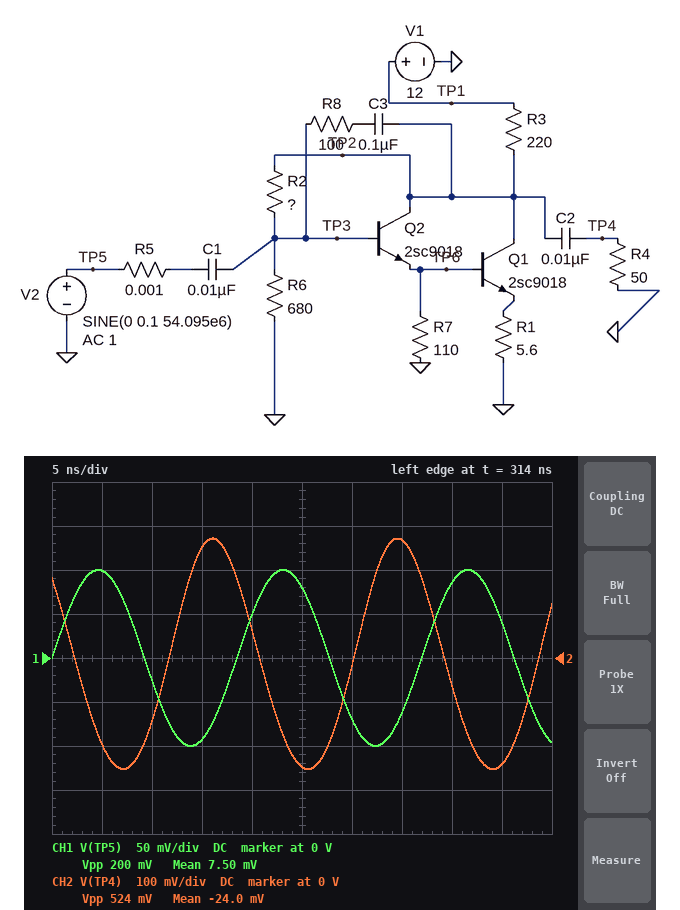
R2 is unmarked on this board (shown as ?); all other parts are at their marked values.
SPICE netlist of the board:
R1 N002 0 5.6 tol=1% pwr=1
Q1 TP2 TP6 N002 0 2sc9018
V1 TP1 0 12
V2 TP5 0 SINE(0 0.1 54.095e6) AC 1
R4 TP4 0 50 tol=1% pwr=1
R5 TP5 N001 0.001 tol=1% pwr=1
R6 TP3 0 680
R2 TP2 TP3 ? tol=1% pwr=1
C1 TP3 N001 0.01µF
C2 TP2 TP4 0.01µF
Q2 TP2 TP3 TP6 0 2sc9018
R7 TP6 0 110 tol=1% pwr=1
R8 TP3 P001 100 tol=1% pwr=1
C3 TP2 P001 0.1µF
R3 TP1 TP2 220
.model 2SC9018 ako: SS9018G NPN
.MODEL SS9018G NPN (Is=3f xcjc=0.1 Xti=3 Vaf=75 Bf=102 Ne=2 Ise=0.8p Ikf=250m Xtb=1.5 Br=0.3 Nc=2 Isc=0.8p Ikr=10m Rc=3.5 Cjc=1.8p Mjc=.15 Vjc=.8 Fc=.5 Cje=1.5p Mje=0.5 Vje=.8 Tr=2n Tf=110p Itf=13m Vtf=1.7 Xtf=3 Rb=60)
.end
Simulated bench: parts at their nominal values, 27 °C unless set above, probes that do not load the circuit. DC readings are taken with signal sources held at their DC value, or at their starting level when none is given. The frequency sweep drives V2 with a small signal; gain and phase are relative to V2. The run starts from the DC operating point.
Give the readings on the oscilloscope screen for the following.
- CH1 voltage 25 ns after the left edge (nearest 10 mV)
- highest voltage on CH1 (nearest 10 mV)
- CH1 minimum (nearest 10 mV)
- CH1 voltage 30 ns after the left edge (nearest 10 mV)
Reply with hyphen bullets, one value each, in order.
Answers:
- 80 mV
- 100 mV
- -100 mV
- -70 mV
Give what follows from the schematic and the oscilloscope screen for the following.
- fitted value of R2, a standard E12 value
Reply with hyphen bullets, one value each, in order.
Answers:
- 390 Ω
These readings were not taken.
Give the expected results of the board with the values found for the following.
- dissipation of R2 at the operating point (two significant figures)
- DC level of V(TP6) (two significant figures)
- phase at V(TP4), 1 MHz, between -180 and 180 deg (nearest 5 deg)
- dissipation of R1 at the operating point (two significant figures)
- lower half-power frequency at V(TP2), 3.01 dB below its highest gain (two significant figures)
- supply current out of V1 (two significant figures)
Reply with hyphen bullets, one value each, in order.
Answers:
- 2.7 mW
- 970 mV
- -125 deg
- 5.3 mW
- 740 kHz
- 42 mA
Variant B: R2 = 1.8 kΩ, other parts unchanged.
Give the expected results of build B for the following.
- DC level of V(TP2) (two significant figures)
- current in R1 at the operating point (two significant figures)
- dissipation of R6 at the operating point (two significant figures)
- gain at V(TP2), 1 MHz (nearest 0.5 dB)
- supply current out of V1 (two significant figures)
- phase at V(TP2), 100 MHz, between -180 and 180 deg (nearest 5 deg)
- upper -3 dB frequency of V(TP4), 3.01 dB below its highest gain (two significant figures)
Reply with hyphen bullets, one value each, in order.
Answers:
- 6.0 V
- 17 mA
- 3.8 mW
- 9.5 dB
- 27 mA
- 135 deg
- 140 MHz
